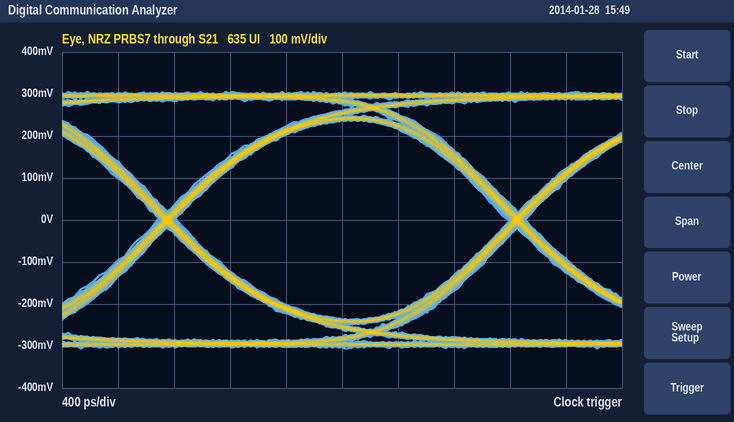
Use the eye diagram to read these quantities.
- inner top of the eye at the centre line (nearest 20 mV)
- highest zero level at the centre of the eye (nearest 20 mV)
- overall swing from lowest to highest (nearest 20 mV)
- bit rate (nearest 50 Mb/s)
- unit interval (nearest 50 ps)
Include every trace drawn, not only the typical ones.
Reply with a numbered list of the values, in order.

1. 240 mV
2. -240 mV
3. 620 mV
4. 400 Mb/s
5. 2.50 ns
